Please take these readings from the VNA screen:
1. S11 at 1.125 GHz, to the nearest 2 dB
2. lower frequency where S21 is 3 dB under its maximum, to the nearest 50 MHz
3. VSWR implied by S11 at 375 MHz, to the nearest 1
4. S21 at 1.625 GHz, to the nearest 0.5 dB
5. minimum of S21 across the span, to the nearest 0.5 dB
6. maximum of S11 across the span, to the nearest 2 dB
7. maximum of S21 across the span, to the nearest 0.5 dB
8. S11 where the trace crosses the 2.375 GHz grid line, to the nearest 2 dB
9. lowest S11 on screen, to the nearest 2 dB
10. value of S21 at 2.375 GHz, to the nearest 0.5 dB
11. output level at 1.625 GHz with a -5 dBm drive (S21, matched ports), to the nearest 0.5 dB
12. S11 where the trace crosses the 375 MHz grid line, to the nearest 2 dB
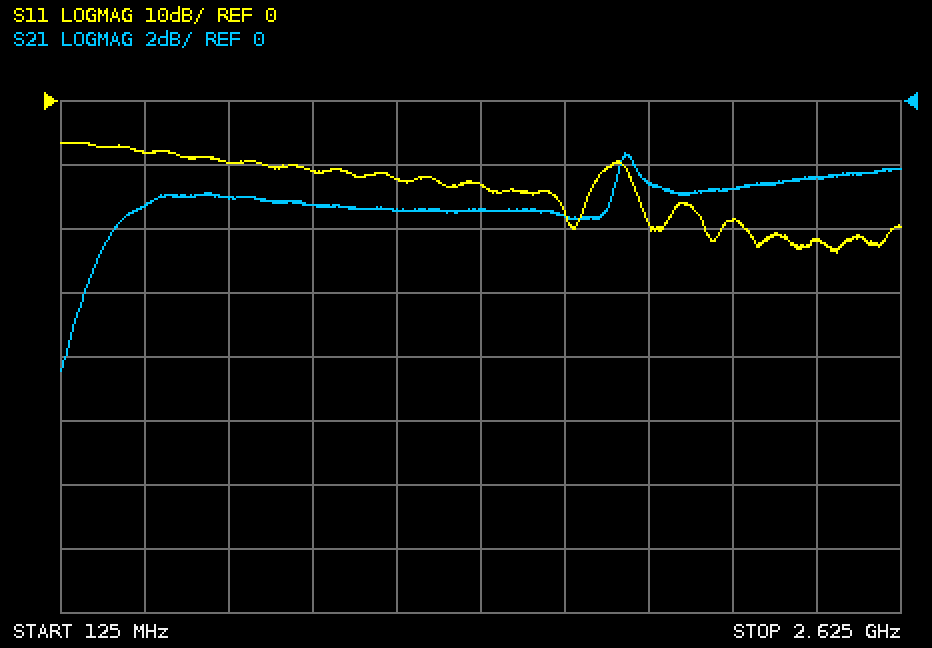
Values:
-12 dB
250 MHz
2
-3.5 dB
-8.5 dB
-6 dB
-1.5 dB
-22 dB
-24 dB
-2.5 dB
-8.5 dBm
-8 dB
